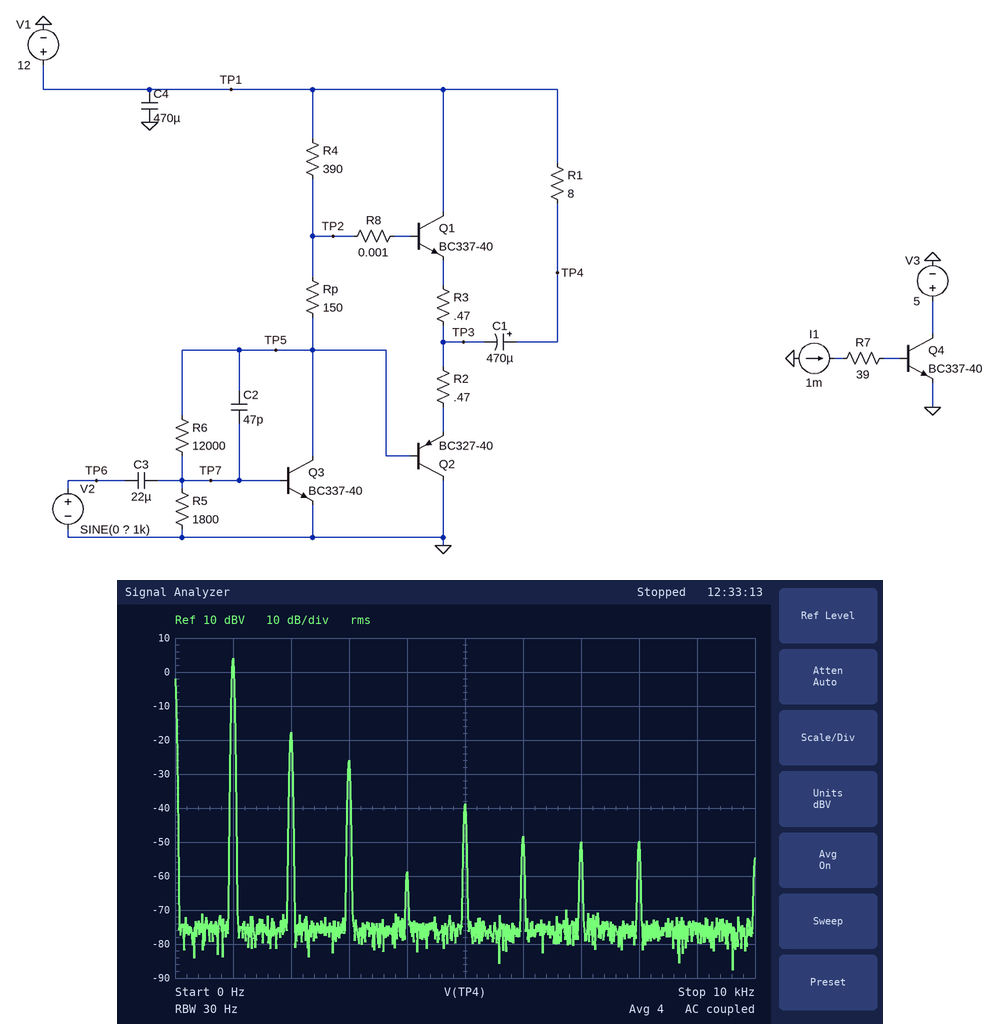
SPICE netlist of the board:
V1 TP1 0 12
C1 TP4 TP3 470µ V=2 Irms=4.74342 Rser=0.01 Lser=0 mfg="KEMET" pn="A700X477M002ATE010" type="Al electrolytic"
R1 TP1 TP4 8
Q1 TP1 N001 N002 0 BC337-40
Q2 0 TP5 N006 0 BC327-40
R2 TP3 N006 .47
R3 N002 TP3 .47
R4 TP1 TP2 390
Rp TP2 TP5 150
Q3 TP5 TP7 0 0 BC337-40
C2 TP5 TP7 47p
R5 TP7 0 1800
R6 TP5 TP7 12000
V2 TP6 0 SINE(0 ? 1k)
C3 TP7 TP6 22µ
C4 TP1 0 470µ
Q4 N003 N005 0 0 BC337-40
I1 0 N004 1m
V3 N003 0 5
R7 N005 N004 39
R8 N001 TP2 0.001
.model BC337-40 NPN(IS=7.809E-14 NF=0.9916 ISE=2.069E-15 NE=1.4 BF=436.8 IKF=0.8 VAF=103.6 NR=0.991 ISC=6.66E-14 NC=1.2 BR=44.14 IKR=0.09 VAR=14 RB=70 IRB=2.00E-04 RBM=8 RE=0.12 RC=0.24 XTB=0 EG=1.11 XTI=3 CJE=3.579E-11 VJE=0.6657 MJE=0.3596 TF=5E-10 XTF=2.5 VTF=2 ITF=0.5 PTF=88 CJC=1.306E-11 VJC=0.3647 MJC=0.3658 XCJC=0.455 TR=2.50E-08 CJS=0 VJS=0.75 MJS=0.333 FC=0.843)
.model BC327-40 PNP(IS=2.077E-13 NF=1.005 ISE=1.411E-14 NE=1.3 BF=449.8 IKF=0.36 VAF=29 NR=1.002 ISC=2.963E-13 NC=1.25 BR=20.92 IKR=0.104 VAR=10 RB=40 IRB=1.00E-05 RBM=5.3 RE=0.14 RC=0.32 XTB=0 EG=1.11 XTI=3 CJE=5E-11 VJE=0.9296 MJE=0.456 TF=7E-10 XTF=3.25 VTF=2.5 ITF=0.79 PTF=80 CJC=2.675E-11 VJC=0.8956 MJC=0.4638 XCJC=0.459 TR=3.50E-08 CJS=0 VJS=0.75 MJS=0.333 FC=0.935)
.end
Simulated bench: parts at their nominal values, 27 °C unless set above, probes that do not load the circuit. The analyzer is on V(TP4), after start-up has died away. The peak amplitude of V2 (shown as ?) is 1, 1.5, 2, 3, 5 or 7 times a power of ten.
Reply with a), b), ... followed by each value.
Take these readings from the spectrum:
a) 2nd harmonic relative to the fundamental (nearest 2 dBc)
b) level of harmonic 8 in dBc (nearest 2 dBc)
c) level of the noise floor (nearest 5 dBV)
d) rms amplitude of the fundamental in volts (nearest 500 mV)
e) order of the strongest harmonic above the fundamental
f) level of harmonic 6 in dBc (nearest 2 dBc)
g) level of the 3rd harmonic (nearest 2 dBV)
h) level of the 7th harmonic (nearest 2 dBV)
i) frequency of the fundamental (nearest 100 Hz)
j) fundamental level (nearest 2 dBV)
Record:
a) -22 dBc
b) -54 dBc
c) -75 dBV
d) 1.5 V
e) 2
f) -52 dBc
g) -26 dBV
h) -50 dBV
i) 1.0 kHz
j) 4 dBV
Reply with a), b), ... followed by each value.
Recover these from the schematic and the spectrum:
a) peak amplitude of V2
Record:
a) 20 mV
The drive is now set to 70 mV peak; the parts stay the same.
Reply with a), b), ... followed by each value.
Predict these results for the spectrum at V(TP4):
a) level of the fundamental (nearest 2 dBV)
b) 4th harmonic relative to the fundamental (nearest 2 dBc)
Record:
a) 10 dBV
b) -20 dBc
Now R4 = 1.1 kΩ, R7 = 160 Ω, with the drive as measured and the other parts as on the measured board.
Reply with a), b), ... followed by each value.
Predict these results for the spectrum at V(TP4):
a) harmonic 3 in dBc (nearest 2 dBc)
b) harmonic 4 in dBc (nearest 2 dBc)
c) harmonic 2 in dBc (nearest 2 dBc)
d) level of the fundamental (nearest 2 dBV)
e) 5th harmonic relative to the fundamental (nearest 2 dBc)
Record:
a) -32 dBc
b) -54 dBc
c) -16 dBc
d) 4 dBV
e) -36 dBc
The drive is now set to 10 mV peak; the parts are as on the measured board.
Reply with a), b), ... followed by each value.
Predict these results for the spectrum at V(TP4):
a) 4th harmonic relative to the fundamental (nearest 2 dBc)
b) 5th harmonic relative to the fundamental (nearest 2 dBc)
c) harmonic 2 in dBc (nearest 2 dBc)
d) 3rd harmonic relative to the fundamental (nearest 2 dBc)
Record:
a) -44 dBc
b) -54 dBc
c) -32 dBc
d) -38 dBc
